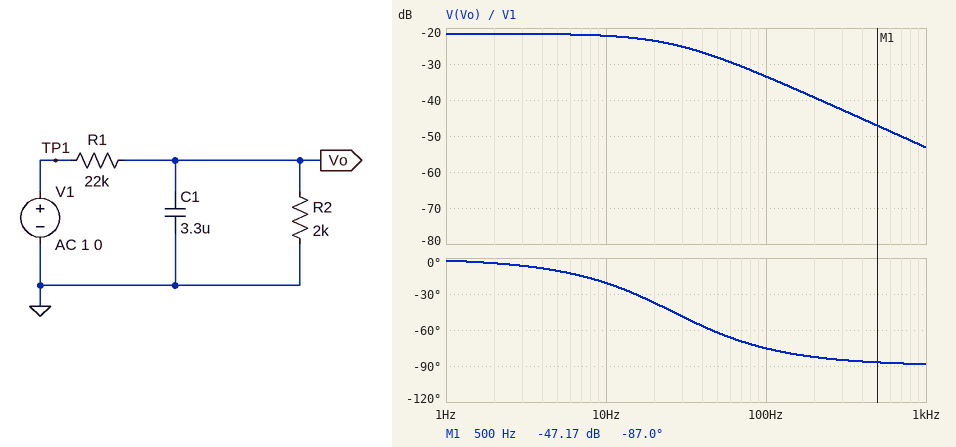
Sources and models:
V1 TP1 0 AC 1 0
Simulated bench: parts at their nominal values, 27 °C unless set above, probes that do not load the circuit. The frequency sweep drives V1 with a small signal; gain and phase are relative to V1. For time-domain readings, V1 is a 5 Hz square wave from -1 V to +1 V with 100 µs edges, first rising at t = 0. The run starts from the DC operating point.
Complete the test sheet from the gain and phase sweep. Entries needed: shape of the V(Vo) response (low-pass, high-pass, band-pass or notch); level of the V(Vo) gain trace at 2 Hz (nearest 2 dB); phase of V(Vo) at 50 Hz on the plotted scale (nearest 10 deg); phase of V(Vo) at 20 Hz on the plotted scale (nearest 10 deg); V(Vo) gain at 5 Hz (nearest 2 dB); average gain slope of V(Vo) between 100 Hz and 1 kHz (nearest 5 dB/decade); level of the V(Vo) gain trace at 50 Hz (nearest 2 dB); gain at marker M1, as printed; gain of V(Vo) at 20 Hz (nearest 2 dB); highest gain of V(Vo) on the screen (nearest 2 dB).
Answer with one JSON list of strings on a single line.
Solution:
["low-pass", "-22 dB", "-60 deg", "-40 deg", "-22 dB", "-20 dB/decade", "-28 dB", "-47.17 dB", "-24 dB", "-22 dB"]
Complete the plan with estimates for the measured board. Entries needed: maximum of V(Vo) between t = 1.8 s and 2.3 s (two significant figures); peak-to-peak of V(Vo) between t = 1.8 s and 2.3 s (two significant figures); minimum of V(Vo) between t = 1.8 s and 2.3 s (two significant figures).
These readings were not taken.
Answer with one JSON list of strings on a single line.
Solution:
["83 mV", "170 mV", "-83 mV"]
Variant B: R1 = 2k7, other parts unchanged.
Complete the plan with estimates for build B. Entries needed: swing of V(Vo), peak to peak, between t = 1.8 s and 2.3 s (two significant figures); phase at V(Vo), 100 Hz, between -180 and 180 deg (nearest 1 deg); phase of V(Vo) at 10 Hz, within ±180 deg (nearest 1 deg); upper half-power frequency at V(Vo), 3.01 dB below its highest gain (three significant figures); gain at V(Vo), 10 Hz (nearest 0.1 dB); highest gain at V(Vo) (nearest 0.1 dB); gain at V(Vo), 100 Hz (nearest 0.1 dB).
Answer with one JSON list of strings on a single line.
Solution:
["850 mV", "-67 deg", "-13 deg", "42.0 Hz", "-7.7 dB", "-7.4 dB", "-15.7 dB"]
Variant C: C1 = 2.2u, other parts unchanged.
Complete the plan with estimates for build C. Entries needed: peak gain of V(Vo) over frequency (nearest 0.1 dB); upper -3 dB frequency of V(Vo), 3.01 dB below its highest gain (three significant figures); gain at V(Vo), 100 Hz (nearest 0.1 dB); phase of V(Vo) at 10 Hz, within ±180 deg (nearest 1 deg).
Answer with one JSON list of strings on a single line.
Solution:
["-21.6 dB", "39.5 Hz", "-30.3 dB", "-14 deg"]
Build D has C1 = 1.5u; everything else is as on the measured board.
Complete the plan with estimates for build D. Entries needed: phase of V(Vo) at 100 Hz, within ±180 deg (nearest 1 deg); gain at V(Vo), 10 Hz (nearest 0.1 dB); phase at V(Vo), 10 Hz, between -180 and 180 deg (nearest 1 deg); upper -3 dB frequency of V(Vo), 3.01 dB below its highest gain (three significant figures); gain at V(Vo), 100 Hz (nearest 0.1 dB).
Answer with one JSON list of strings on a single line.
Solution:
["-60 deg", "-21.7 dB", "-10 deg", "57.9 Hz", "-27.6 dB"]
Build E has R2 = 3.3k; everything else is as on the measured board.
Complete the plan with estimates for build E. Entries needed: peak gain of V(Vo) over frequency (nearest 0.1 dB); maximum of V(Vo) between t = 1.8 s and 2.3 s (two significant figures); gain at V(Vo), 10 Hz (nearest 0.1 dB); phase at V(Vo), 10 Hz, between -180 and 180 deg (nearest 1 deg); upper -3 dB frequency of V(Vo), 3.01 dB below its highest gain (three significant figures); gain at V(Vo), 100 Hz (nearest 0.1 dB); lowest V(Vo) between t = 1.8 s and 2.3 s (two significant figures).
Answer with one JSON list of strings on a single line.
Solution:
["-17.7 dB", "130 mV", "-19.0 dB", "-31 deg", "16.8 Hz", "-33.3 dB", "-130 mV"]
